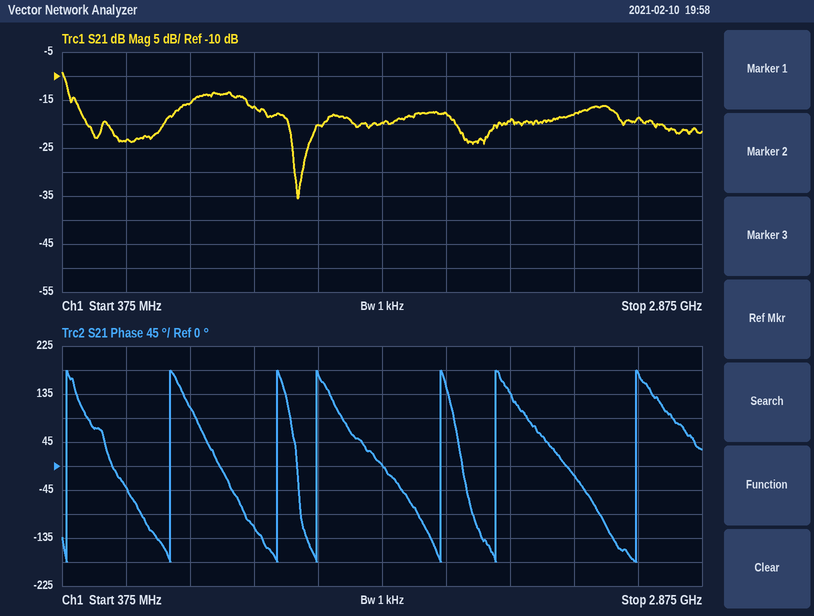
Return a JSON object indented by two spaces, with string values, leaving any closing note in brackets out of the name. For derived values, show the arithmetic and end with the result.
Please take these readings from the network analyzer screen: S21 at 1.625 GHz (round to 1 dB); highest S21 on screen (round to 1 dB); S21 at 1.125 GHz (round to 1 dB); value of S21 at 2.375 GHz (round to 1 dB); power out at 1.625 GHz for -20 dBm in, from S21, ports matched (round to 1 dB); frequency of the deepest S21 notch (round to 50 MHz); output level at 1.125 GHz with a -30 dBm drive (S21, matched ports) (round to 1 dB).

{
  "S21 at 1.625 GHz": "-20 dB",
  "highest S21 on screen": "-9 dB",
  "S21 at 1.125 GHz": "-16 dB",
  "value of S21 at 2.375 GHz": "-18 dB",
  "power out at 1.625 GHz for -20 dBm in, from S21, ports matched": "-20 dBm + (-20 dB) = -40 dBm",
  "frequency of the deepest S21 notch": "1.30 GHz",
  "output level at 1.125 GHz with a -30 dBm drive (S21, matched ports)": "-30 dBm + (-16 dB) = -46 dBm"
}
